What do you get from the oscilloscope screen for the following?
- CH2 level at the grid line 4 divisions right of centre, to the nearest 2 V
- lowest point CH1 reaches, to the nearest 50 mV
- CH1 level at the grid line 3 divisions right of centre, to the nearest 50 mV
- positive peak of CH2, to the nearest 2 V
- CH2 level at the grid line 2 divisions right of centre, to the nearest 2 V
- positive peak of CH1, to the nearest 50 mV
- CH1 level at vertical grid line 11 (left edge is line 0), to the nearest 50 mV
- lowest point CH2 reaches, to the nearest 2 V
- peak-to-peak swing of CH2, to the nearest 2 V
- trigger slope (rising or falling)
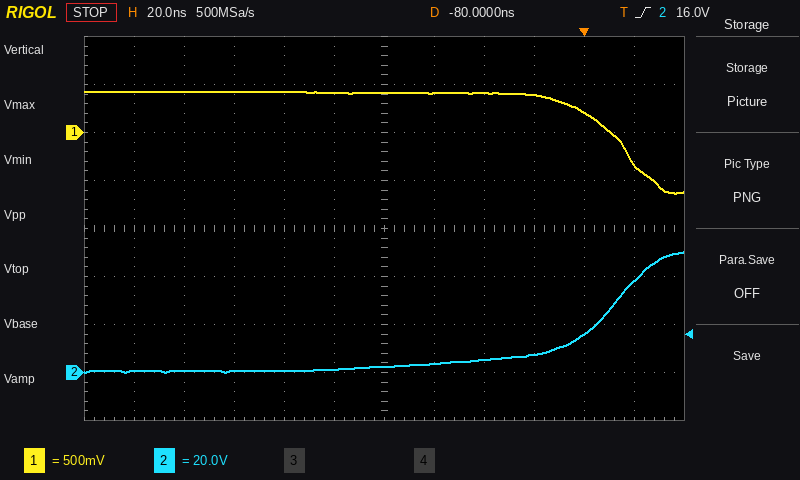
16 V
-650 mV
400 mV
50 V
6 V
450 mV
-350 mV
0 V
50 V
rising
